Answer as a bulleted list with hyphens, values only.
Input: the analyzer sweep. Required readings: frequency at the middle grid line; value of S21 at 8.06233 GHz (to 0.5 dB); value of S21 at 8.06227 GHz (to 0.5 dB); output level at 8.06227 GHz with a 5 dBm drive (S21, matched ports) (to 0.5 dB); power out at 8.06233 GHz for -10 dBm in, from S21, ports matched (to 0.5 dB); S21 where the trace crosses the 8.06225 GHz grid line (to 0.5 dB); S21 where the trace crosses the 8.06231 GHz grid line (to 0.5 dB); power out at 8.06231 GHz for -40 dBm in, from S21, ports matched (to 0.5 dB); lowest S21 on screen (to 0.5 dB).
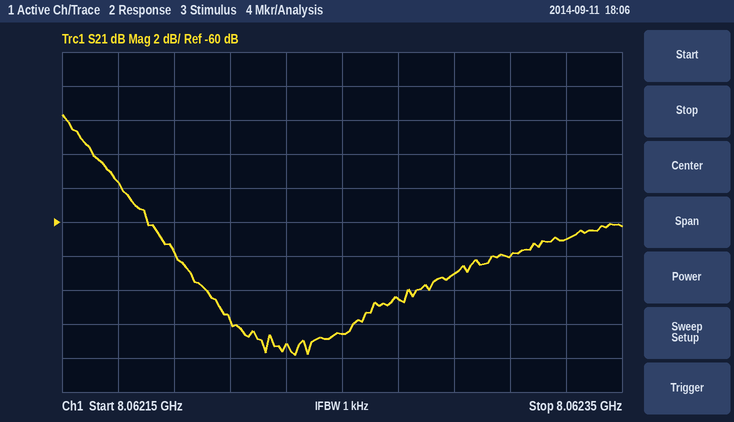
- 8.06225 GHz
- -61.0 dB
- -64.5 dB
- -59.5 dBm
- -71.0 dBm
- -66.5 dB
- -62.0 dB
- -102.0 dBm
- -68.0 dB
